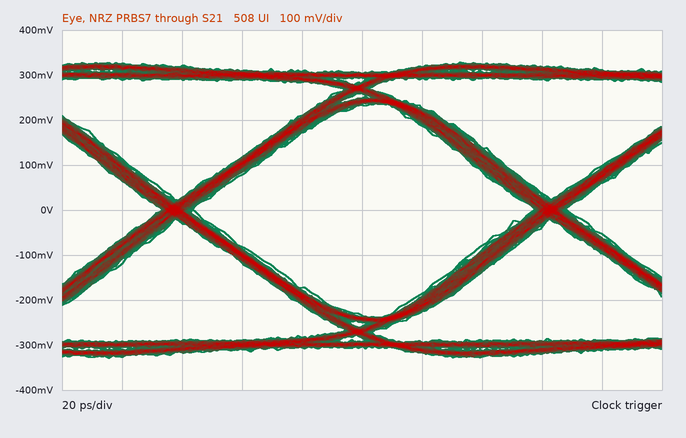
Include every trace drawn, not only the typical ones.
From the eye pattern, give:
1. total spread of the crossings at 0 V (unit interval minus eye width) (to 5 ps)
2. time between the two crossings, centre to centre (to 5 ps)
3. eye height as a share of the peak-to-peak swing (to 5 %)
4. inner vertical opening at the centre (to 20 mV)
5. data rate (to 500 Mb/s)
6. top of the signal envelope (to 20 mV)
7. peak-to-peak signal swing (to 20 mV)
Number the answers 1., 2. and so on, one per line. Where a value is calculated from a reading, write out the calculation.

1. 10 ps
2. 125 ps
3. 460 mV / 660 mV ≈ 70 %
4. 460 mV
5. 8.0 Gb/s
6. 320 mV
7. 660 mV
